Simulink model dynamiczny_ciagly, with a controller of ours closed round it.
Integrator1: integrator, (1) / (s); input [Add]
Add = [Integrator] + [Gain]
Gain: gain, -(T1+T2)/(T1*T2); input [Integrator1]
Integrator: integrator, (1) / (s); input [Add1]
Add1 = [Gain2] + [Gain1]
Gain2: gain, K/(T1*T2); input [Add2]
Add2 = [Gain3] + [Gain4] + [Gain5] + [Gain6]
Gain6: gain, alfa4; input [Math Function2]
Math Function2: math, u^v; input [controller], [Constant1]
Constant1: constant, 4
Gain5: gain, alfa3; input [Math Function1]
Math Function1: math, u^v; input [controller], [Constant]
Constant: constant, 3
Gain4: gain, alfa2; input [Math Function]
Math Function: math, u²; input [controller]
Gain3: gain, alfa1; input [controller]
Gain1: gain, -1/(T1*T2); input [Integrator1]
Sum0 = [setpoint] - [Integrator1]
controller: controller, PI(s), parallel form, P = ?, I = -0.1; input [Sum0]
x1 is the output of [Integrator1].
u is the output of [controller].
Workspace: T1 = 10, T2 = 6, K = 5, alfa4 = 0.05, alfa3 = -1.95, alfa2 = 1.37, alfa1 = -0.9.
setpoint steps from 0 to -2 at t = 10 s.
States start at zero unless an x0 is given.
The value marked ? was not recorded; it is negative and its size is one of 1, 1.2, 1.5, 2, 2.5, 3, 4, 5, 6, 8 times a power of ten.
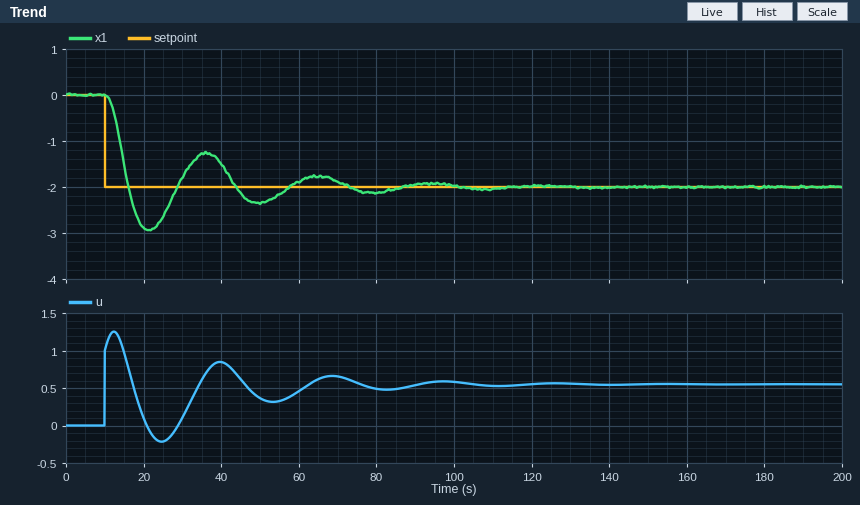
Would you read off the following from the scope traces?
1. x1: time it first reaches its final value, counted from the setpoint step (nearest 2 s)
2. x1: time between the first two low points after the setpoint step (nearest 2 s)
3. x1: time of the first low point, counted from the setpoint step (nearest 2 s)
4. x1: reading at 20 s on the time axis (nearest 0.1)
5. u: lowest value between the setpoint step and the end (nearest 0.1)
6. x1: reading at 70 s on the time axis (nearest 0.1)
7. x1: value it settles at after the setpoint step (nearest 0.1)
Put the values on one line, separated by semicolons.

6 s; 28 s; 12 s; -2.9; -0.2; -1.9; -2.0
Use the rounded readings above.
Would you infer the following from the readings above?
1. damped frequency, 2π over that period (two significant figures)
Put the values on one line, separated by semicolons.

0.22 rad/s
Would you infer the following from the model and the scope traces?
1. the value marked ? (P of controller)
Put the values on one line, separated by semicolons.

-0.5
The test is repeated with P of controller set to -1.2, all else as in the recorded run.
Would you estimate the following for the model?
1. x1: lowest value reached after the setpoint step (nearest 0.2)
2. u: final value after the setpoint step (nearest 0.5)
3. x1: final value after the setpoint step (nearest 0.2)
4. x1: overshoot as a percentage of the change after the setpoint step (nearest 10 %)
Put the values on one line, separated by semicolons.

-3.2; 0.5; -2.0; 60 %
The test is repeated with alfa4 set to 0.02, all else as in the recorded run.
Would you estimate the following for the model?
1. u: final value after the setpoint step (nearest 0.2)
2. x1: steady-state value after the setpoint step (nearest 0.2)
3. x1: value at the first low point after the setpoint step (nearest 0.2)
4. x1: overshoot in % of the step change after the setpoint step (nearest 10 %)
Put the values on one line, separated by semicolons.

0.6; -2.0; -3.0; 50 %
